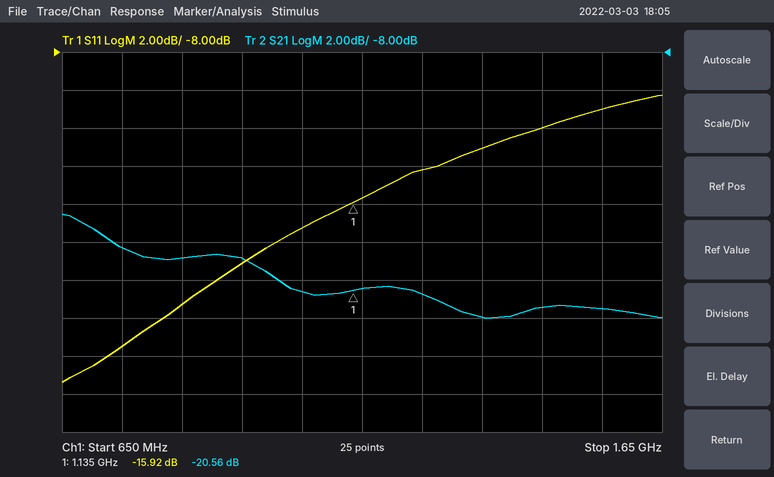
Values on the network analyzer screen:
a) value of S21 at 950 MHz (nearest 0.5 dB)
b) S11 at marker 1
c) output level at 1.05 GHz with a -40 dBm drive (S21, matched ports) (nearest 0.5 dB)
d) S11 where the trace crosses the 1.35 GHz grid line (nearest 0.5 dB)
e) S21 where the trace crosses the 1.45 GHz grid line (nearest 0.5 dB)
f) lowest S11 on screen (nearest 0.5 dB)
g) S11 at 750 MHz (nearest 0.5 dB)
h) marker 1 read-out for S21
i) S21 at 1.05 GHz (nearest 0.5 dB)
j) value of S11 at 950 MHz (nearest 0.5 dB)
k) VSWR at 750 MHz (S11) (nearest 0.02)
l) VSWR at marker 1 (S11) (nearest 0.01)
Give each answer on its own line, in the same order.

-19.0 dB
-15.92 dB
-60.5 dBm
-13.0 dB
-21.5 dB
-25.5 dB
-23.5 dB
-20.56 dB
-20.5 dB
-19.0 dB
1.14
1.38
